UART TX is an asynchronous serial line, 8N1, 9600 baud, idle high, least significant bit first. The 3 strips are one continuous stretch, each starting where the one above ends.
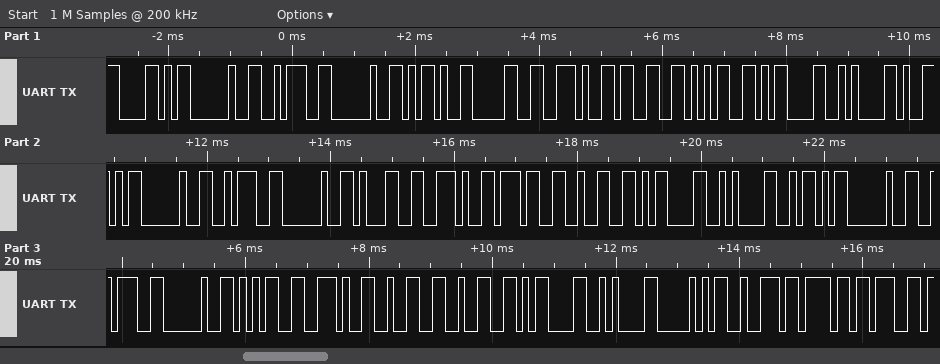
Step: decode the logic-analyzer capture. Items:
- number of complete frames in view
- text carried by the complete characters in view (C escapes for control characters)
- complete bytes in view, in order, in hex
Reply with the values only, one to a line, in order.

35
"X : -0.35\r\nY : 1.72\r\nZ : 5.22\r\nProg"
58 20 3A 20 2D 30 2E 33 35 0D 0A 59 20 3A 20 31 2E 37 32 0D 0A 5A 20 3A 20 35 2E 32 32 0D 0A 50 72 6F 67
